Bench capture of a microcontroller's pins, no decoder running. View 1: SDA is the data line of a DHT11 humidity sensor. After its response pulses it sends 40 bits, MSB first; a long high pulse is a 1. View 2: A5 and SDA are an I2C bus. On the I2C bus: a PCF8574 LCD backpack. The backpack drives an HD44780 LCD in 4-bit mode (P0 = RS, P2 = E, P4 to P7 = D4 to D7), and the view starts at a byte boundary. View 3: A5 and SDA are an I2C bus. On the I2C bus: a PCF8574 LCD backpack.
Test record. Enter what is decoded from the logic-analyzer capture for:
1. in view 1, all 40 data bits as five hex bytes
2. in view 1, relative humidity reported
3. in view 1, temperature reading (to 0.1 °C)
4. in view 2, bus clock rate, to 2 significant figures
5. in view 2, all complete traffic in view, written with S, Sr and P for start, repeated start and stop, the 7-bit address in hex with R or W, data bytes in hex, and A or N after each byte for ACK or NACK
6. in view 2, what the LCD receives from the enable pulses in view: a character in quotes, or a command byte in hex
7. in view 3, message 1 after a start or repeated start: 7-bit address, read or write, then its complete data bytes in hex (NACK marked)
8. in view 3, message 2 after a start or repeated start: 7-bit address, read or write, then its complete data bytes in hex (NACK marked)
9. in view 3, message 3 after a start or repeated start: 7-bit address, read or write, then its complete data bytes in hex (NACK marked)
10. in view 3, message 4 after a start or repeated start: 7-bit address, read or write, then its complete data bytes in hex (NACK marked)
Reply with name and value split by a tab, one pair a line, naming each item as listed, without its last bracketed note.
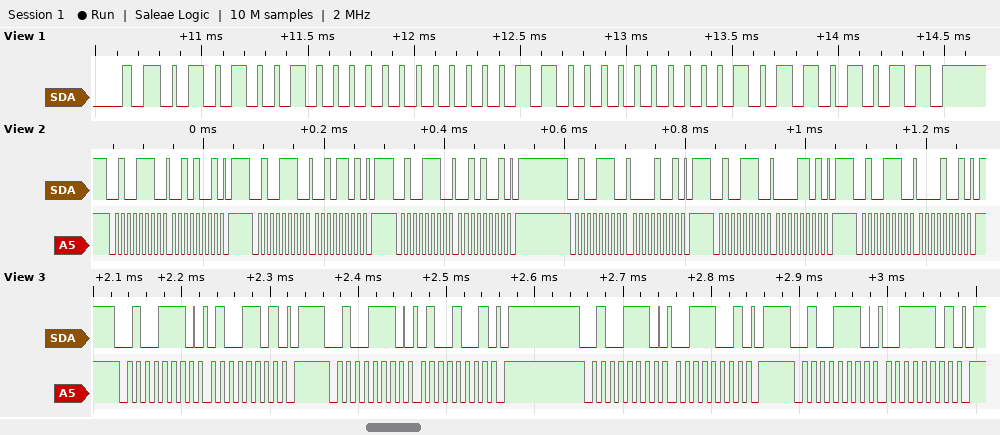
in view 1, all 40 data bits as five hex bytes	52 00 18 01 6B
in view 1, relative humidity reported	82 %
in view 1, temperature reading	24.1 °C
in view 2, bus clock rate, to 2 significant figures	100 kHz
in view 2, all complete traffic in view, written with S, Sr and P for start, repeated start and stop, the 7-bit address in hex with R or W, data bytes in hex, and A or N after each byte for ACK or NACK	S 27W A 29 A P S 27W A 2D A P S 27W A 29 A P S 27W A 09 A P S 27W A 0D A P S 27W A 09 A P
in view 2, what the LCD receives from the enable pulses in view: a character in quotes, or a command byte in hex	' '
in view 3, message 1 after a start or repeated start: 7-bit address, read or write, then its complete data bytes in hex	0x27 write: 4D
in view 3, message 2 after a start or repeated start: 7-bit address, read or write, then its complete data bytes in hex	0x27 write: 49
in view 3, message 3 after a start or repeated start: 7-bit address, read or write, then its complete data bytes in hex	0x27 write: 39
in view 3, message 4 after a start or repeated start: 7-bit address, read or write, then its complete data bytes in hex	0x27 write: 3D
